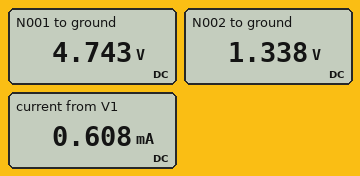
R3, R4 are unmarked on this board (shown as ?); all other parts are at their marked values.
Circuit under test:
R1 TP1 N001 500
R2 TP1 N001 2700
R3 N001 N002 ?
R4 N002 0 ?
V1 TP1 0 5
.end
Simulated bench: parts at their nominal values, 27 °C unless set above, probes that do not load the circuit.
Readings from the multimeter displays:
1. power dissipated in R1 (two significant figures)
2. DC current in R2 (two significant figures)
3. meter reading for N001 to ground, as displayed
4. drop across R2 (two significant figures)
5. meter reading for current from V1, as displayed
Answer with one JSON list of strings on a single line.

["130 µW", "95 µA", "4.743 V", "260 mV", "0.608 mA"]
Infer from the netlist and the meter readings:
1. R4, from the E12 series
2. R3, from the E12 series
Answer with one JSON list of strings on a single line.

["2.2 kΩ", "5.6 kΩ"]
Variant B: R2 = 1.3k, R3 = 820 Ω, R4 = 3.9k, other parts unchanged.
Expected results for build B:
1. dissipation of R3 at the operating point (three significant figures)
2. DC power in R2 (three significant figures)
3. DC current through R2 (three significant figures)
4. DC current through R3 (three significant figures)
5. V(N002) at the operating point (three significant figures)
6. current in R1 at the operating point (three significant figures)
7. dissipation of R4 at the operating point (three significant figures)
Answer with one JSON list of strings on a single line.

["794 µW", "97.1 µW", "273 µA", "984 µA", "3.84 V", "711 µA", "3.78 mW"]
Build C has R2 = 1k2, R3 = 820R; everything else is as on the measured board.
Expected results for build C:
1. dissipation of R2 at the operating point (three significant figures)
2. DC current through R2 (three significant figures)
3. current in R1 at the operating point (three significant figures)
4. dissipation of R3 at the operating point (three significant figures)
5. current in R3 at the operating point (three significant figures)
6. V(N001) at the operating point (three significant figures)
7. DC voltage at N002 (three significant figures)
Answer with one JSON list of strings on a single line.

["228 µW", "436 µA", "1.05 mA", "1.80 mW", "1.48 mA", "4.48 V", "3.26 V"]
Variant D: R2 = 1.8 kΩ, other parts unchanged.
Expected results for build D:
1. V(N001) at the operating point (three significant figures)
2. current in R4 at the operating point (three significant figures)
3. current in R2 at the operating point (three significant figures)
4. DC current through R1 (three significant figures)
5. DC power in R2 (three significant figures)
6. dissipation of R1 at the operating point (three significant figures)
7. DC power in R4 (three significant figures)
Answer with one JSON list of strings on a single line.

["4.76 V", "610 µA", "133 µA", "478 µA", "31.7 µW", "114 µW", "820 µW"]
